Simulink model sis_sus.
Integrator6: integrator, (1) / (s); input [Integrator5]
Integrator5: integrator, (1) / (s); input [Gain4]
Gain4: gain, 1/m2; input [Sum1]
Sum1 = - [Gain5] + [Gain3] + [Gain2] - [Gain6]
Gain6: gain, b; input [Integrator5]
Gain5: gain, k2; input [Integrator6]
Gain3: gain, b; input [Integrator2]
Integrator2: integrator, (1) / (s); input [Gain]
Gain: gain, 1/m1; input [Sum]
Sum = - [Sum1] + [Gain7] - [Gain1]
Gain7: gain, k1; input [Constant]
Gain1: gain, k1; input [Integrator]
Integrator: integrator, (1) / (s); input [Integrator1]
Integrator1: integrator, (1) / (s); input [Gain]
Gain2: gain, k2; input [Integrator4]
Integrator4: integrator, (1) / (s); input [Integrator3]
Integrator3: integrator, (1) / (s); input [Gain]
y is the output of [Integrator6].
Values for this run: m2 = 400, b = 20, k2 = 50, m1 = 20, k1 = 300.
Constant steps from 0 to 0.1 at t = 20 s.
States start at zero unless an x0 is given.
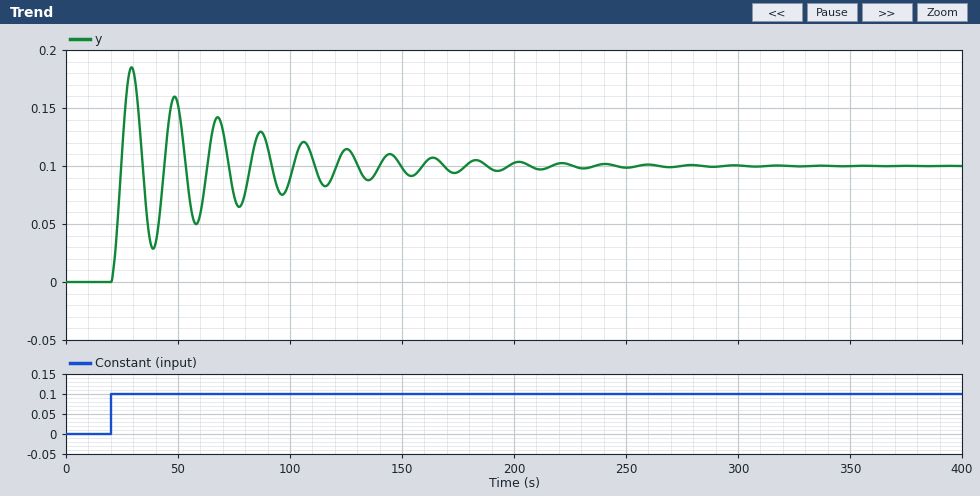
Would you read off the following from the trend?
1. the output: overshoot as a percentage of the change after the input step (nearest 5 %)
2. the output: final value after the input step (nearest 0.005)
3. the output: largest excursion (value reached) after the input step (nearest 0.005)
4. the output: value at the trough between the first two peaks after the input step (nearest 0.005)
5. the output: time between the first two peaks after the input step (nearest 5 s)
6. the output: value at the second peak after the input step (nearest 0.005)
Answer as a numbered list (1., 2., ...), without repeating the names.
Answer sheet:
1. 85 %
2. 0.100
3. 0.185
4. 0.030
5. 20 s
6. 0.160
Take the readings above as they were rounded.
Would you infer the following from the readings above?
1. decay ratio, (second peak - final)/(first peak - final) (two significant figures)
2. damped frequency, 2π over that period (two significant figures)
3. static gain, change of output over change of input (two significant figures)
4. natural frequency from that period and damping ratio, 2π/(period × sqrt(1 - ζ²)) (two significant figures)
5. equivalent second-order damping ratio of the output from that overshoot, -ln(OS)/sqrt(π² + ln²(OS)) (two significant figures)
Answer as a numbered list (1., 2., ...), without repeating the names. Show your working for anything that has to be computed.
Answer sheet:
1. (0.16 - 0.1) / (0.185 - 0.1) = 0.71
2. 2π / 20 = 0.31 rad/s
3. (0.1 - 0) / (0.1 - 0) = 1.0
4. 2π / (20 × sqrt(1 - 0.052²)) = 0.31 rad/s
5. ln(0.85) = -0.163; 0.163 / sqrt(9.870 + 0.026) = 0.052
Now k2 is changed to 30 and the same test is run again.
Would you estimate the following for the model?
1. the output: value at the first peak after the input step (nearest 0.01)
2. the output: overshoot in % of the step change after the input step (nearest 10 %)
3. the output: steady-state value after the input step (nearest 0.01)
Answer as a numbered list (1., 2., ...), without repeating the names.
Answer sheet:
1. 0.18
2. 80 %
3. 0.10
